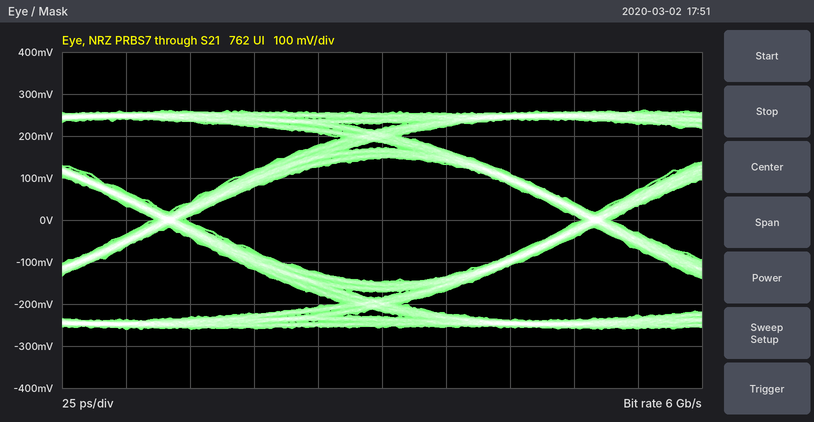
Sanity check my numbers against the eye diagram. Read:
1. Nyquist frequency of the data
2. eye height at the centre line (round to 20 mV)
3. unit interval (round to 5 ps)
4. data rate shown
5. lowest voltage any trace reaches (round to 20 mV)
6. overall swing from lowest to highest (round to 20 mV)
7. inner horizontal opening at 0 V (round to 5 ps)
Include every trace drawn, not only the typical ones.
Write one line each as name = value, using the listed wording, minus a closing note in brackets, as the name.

Nyquist frequency of the data = 3 GHz
eye height at the centre line = 300 mV
unit interval = 165 ps
data rate shown = 6 Gb/s
lowest voltage any trace reaches = -260 mV
overall swing from lowest to highest = 520 mV
inner horizontal opening at 0 V = 155 ps
